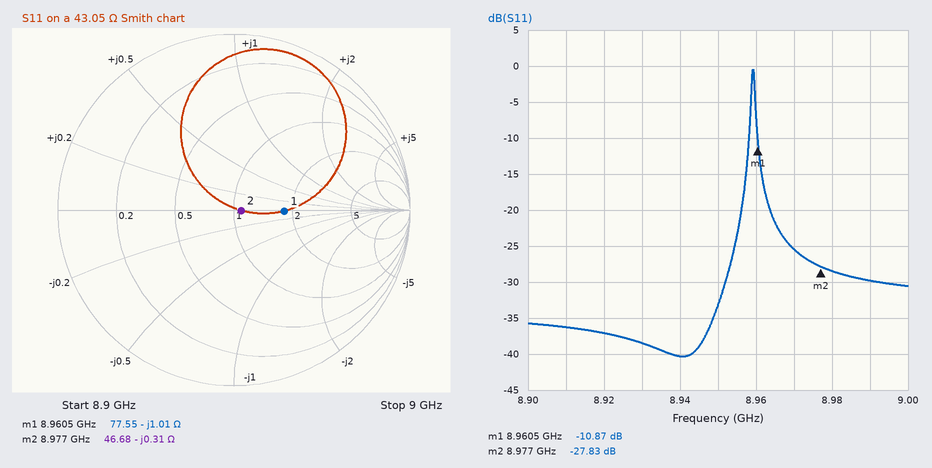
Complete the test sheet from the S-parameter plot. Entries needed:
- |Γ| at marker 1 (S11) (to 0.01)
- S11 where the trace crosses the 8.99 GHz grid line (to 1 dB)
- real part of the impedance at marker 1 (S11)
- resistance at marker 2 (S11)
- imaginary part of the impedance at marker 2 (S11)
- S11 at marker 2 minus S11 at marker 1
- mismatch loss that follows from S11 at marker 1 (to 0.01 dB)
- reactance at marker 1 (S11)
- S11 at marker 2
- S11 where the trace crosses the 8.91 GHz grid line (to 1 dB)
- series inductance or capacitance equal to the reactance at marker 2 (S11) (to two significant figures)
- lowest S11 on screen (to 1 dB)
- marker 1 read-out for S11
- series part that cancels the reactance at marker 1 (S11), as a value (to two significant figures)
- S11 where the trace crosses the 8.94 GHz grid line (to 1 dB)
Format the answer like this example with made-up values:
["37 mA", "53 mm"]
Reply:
["0.29", "-30 dB", "77.55 Ω", "46.68 Ω", "-0.31 Ω", "-16.96 dB", "0.37 dB", "-1.01 Ω", "-27.83 dB", "-36 dB", "57 pF", "-40 dB", "-10.87 dB", "18 pH", "-40 dB"]
